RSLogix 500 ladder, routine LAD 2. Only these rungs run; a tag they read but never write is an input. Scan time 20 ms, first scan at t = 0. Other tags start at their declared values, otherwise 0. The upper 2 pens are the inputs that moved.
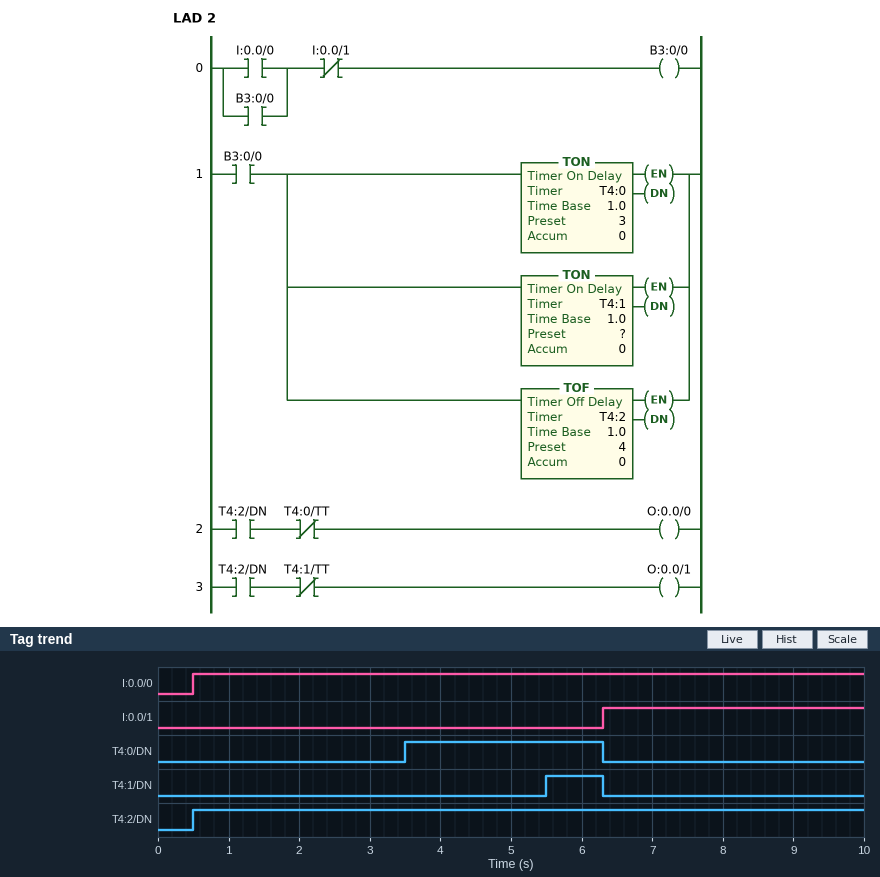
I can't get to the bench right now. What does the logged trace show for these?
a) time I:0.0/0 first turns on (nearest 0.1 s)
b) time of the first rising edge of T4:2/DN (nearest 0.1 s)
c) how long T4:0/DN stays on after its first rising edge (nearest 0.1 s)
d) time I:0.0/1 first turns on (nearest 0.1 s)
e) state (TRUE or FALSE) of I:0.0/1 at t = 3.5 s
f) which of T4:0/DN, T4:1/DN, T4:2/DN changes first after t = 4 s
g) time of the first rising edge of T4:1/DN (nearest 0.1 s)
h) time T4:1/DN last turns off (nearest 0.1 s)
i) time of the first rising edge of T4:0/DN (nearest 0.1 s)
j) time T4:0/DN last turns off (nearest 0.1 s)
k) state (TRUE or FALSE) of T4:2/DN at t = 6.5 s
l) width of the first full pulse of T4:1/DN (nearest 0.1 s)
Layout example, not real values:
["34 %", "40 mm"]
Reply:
["0.5 s", "0.5 s", "2.8 s", "6.3 s", "FALSE", "T4:1/DN", "5.5 s", "6.3 s", "3.5 s", "6.3 s", "TRUE", "0.8 s"]
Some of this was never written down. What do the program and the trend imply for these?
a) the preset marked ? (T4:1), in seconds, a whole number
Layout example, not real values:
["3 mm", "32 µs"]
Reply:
["5 s"]
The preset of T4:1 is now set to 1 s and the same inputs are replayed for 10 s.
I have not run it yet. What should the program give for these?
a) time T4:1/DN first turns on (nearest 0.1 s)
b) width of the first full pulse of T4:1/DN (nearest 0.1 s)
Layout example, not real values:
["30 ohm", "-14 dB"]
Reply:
["1.5 s", "4.8 s"]
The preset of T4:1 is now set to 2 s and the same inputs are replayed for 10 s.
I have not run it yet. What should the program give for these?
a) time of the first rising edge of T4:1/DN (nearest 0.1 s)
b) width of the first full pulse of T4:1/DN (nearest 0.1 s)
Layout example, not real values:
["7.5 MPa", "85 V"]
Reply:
["2.5 s", "3.8 s"]
